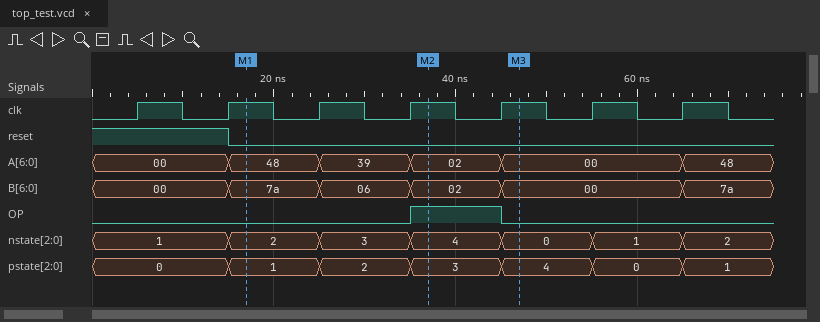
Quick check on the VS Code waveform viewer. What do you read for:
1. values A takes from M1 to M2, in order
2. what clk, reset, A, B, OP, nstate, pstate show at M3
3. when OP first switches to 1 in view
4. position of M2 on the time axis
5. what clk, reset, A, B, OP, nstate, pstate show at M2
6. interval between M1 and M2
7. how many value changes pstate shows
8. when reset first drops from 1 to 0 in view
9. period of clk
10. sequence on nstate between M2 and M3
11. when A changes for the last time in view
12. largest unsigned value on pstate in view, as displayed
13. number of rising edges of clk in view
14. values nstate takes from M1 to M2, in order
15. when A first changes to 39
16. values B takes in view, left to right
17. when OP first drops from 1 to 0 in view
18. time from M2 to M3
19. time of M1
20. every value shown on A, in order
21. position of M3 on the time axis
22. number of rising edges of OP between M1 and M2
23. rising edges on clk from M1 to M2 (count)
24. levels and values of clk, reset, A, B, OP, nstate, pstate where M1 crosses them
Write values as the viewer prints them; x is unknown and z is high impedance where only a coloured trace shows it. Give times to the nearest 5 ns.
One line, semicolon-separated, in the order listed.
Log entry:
48, 39, 02; clk=1, reset=0, A=00, B=00, OP=0, nstate=0, pstate=4; 35 ns; 35 ns; clk=1, reset=0, A=02, B=02, OP=1, nstate=4, pstate=3; 20 ns; 6; 15 ns; 10 ns; 4, 0; 65 ns; 4; 7; 2, 3, 4; 25 ns; 00, 7a, 06, 02, 00, 7a; 45 ns; 10 ns; 15 ns; 00, 48, 39, 02, 00, 48; 45 ns; 1; 2; clk=1, reset=0, A=48, B=7a, OP=0, nstate=2, pstate=1
